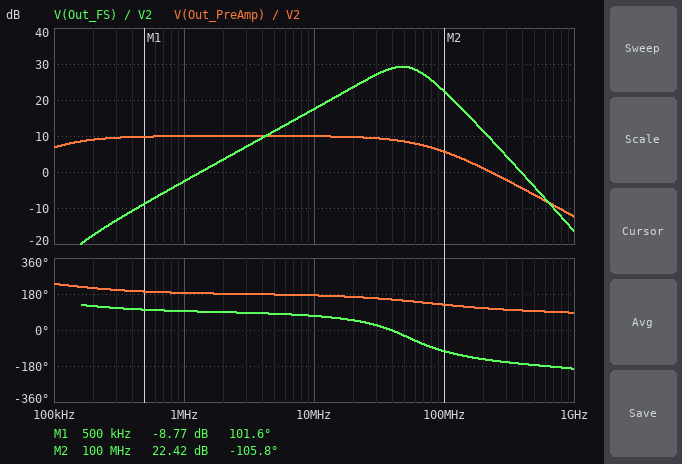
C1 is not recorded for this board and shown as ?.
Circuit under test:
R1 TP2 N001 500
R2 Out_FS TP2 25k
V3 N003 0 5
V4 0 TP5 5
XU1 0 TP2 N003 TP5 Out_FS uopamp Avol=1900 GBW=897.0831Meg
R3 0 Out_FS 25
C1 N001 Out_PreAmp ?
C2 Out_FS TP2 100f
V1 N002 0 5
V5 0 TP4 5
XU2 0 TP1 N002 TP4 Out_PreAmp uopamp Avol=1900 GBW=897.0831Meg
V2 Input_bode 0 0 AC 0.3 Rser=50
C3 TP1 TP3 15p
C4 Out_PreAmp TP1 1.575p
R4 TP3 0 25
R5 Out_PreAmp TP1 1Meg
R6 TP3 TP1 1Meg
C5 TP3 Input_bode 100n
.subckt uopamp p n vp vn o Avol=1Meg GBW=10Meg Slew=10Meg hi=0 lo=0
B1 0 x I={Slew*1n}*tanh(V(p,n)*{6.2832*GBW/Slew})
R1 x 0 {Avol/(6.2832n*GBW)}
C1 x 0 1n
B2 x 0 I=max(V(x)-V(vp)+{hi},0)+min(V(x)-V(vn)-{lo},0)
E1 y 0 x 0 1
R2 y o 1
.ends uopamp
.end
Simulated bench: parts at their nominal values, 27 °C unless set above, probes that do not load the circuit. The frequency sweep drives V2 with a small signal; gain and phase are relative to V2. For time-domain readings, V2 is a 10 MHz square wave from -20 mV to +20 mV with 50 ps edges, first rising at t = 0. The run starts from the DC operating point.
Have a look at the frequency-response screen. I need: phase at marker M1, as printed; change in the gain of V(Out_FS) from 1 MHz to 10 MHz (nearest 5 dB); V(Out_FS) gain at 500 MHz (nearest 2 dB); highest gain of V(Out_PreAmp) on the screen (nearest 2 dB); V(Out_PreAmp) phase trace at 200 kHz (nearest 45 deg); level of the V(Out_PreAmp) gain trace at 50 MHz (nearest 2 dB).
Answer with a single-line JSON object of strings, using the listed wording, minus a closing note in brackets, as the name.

{"phase at marker M1, as printed": "101.6 deg", "change in the gain of V(Out_FS) from 1 MHz to 10 MHz": "20 dB", "V(Out_FS) gain at 500 MHz": "-4 dB", "highest gain of V(Out_PreAmp) on the screen": "10 dB", "V(Out_PreAmp) phase trace at 200 kHz": "225 deg", "level of the V(Out_PreAmp) gain trace at 50 MHz": "8 dB"}
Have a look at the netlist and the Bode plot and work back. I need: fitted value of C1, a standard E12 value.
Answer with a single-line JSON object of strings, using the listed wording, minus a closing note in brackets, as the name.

{"fitted value of C1, a standard E12 value": "1.5 pF"}
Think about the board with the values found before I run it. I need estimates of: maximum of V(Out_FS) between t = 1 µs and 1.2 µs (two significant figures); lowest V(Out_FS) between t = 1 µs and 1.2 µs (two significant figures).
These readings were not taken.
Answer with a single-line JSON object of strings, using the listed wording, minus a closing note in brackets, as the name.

{"maximum of V(Out_FS) between t = 1 µs and 1.2 µs": "240 mV", "lowest V(Out_FS) between t = 1 µs and 1.2 µs": "-240 mV"}
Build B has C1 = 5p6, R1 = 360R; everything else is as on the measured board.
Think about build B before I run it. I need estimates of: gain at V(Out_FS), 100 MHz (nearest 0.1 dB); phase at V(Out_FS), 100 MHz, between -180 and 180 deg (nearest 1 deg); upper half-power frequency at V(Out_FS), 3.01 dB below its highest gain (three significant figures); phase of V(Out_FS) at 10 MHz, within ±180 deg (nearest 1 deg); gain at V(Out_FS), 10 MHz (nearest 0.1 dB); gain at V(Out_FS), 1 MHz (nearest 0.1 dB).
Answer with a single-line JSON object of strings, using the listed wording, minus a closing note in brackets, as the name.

{"gain at V(Out_FS), 100 MHz": "23.1 dB", "phase at V(Out_FS), 100 MHz, between -180 and 180 deg": "-130 deg", "upper half-power frequency at V(Out_FS), 3.01 dB below its highest gain": "40.7 MHz", "phase of V(Out_FS) at 10 MHz, within ±180 deg": "64 deg", "gain at V(Out_FS), 10 MHz": "29.5 dB", "gain at V(Out_FS), 1 MHz": "8.8 dB"}
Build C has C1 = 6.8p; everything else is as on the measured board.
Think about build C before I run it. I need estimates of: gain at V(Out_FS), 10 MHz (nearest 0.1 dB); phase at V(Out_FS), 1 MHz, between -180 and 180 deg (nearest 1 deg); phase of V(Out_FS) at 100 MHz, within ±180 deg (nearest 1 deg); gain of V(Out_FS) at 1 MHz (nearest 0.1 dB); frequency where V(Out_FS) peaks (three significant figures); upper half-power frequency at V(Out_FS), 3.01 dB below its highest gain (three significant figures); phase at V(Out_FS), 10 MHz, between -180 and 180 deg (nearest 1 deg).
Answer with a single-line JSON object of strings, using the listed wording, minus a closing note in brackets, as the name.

{"gain at V(Out_FS), 10 MHz": "31.2 dB", "phase at V(Out_FS), 1 MHz, between -180 and 180 deg": "93 deg", "phase of V(Out_FS) at 100 MHz, within ±180 deg": "-130 deg", "gain of V(Out_FS) at 1 MHz": "10.5 dB", "frequency where V(Out_FS) peaks": "24.4 MHz", "upper half-power frequency at V(Out_FS), 3.01 dB below its highest gain": "37.7 MHz", "phase at V(Out_FS), 10 MHz, between -180 and 180 deg": "58 deg"}
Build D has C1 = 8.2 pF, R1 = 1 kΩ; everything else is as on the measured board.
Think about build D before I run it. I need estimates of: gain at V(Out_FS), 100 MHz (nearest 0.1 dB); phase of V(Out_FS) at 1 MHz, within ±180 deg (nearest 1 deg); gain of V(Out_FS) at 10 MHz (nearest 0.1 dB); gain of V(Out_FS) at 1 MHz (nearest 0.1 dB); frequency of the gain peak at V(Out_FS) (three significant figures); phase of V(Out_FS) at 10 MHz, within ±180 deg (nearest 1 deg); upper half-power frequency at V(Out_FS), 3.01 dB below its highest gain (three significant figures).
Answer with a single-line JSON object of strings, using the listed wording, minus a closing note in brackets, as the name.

{"gain at V(Out_FS), 100 MHz": "20.4 dB", "phase of V(Out_FS) at 1 MHz, within ±180 deg": "92 deg", "gain of V(Out_FS) at 10 MHz": "31.9 dB", "gain of V(Out_FS) at 1 MHz": "12.1 dB", "frequency of the gain peak at V(Out_FS)": "20.0 MHz", "phase of V(Out_FS) at 10 MHz, within ±180 deg": "41 deg", "upper half-power frequency at V(Out_FS), 3.01 dB below its highest gain": "36.7 MHz"}
